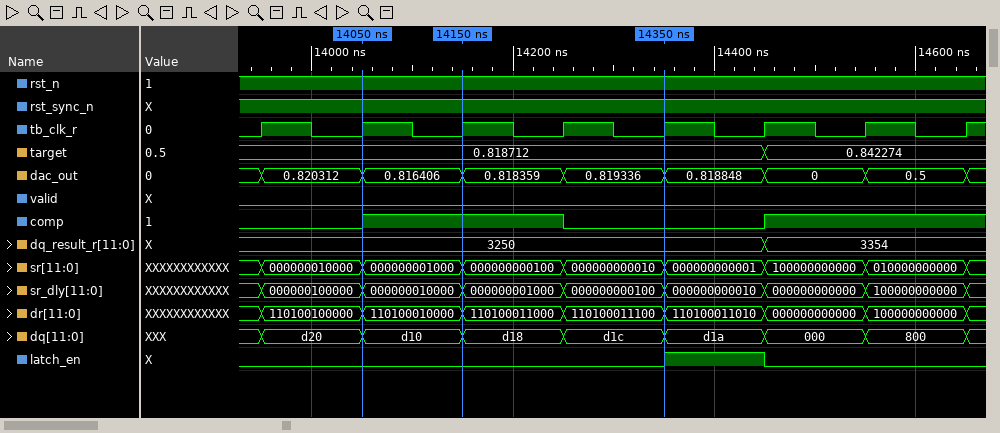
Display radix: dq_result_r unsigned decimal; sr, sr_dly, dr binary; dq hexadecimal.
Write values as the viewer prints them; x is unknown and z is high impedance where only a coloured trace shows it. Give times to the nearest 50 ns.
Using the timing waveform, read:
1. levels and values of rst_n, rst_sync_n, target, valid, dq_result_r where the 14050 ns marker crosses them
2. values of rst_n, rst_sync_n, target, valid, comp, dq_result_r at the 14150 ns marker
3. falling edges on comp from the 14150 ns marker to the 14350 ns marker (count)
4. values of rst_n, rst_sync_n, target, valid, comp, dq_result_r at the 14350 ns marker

rst_n=1, rst_sync_n=1, target=0.818712, valid=0, dq_result_r=3250
rst_n=1, rst_sync_n=1, target=0.818712, valid=0, comp=1, dq_result_r=3250
1
rst_n=1, rst_sync_n=1, target=0.818712, valid=0, comp=0, dq_result_r=3250
